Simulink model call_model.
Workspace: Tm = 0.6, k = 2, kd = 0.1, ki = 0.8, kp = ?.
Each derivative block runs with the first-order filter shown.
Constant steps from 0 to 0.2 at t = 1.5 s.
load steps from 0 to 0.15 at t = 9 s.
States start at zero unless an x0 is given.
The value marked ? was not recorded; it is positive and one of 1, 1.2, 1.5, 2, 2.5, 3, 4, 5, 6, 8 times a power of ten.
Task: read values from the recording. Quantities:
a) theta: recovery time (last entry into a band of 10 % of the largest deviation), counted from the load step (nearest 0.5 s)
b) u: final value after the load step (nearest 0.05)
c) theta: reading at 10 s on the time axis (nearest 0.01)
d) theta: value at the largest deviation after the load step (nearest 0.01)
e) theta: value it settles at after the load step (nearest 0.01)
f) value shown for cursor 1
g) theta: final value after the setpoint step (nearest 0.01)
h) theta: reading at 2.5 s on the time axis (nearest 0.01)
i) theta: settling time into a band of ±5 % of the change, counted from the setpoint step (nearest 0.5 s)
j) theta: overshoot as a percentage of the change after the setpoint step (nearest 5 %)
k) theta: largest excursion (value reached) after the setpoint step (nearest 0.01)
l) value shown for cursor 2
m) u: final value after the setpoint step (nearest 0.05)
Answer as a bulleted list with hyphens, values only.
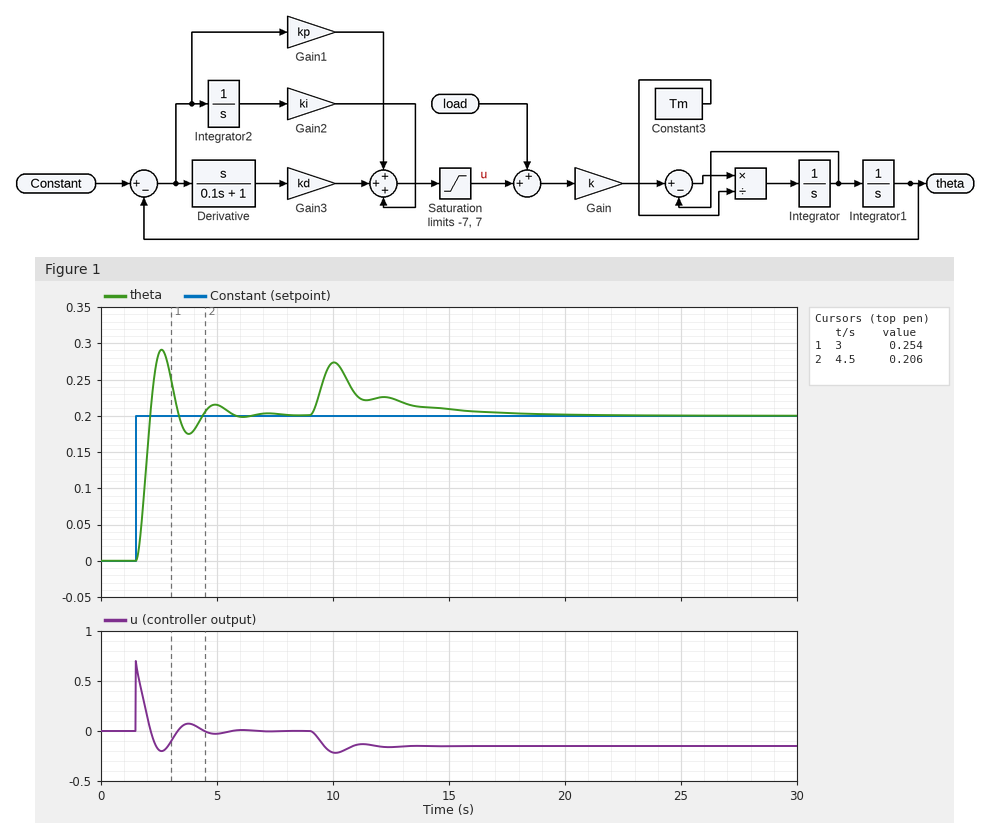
- 6.5 s
- -0.15
- 0.27
- 0.27
- 0.20
- 0.254
- 0.20
- 0.29
- 4.0 s
- 45 %
- 0.29
- 0.206
- 0.00
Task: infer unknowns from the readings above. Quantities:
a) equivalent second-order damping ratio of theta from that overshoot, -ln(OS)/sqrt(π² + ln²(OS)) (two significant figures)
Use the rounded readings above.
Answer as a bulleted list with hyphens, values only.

- 0.25
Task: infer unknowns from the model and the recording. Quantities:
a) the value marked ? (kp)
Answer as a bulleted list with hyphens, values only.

- 2.5
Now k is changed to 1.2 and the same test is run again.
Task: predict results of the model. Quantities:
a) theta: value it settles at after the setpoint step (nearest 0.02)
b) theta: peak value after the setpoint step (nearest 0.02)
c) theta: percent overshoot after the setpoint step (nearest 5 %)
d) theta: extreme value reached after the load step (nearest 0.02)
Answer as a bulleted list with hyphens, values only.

- 0.20
- 0.28
- 40 %
- 0.26
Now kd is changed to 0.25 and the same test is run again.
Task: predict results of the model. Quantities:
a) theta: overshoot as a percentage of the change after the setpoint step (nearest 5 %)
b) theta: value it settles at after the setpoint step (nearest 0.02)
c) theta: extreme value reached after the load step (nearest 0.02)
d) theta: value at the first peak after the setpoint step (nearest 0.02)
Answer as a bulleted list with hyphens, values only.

- 35 %
- 0.20
- 0.26
- 0.28
